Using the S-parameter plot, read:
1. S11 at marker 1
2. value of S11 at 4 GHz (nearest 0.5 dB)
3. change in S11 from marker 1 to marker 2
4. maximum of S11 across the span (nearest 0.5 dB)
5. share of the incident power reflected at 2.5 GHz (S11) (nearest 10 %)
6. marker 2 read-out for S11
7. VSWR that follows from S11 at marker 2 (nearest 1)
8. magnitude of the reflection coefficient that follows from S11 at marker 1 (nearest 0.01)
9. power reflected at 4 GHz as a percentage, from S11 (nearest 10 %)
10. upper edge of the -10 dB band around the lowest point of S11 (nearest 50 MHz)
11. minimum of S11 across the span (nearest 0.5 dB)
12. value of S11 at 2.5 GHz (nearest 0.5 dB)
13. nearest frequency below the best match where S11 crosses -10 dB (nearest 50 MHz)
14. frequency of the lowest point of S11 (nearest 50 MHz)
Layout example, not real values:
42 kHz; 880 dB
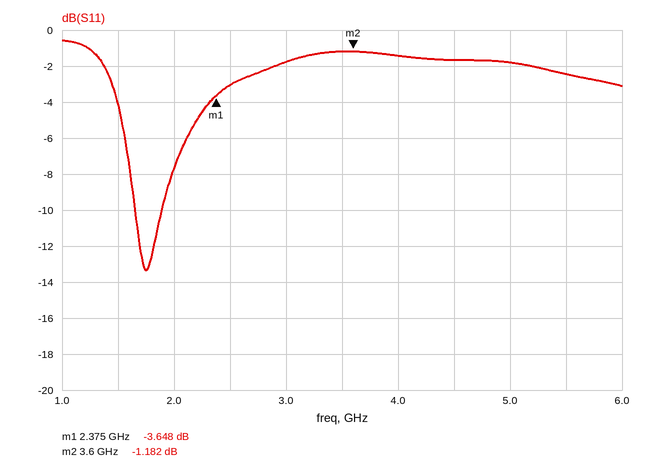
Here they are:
-3.648 dB; -1.5 dB; 2.466 dB; -0.5 dB; 50 %; -1.182 dB; 15; 0.66; 70 %; 1.90 GHz; -13.5 dB; -3.0 dB; 1.65 GHz; 1.75 GHz
